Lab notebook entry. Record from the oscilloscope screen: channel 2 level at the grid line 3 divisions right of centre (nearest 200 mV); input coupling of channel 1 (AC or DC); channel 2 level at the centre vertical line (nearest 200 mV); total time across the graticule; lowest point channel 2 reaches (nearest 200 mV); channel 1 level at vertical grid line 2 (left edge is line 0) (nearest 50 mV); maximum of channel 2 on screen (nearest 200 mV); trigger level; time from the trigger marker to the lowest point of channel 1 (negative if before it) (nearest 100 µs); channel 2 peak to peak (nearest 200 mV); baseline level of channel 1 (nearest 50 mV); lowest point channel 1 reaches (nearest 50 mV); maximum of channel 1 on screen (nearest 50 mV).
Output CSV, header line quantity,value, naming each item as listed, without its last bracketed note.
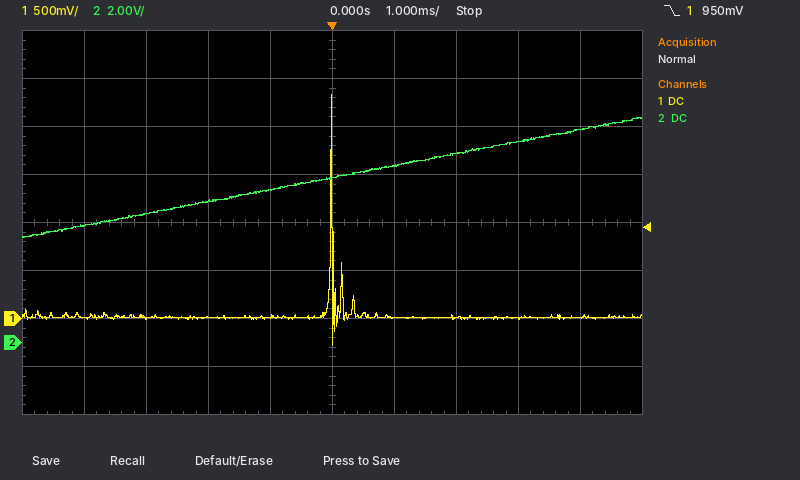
quantity,value
channel 2 level at the grid line 3 divisions right of centre,8.4 V
input coupling of channel 1,DC
channel 2 level at the centre vertical line,6.8 V
total time across the graticule,10 ms
lowest point channel 2 reaches,4.4 V
channel 1 level at vertical grid line 2 (left edge is line 0),0 mV
maximum of channel 2 on screen,9.4 V
trigger level,950 mV
time from the trigger marker to the lowest point of channel 1 (negative if before it),0.0 ms
channel 2 peak to peak,5.0 V
baseline level of channel 1,0 mV
lowest point channel 1 reaches,-300 mV
maximum of channel 1 on screen,2.35 V
